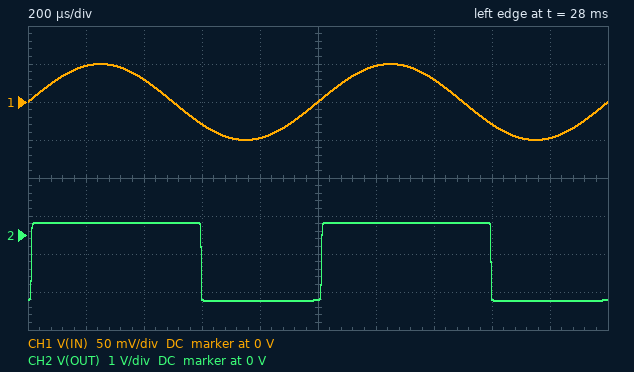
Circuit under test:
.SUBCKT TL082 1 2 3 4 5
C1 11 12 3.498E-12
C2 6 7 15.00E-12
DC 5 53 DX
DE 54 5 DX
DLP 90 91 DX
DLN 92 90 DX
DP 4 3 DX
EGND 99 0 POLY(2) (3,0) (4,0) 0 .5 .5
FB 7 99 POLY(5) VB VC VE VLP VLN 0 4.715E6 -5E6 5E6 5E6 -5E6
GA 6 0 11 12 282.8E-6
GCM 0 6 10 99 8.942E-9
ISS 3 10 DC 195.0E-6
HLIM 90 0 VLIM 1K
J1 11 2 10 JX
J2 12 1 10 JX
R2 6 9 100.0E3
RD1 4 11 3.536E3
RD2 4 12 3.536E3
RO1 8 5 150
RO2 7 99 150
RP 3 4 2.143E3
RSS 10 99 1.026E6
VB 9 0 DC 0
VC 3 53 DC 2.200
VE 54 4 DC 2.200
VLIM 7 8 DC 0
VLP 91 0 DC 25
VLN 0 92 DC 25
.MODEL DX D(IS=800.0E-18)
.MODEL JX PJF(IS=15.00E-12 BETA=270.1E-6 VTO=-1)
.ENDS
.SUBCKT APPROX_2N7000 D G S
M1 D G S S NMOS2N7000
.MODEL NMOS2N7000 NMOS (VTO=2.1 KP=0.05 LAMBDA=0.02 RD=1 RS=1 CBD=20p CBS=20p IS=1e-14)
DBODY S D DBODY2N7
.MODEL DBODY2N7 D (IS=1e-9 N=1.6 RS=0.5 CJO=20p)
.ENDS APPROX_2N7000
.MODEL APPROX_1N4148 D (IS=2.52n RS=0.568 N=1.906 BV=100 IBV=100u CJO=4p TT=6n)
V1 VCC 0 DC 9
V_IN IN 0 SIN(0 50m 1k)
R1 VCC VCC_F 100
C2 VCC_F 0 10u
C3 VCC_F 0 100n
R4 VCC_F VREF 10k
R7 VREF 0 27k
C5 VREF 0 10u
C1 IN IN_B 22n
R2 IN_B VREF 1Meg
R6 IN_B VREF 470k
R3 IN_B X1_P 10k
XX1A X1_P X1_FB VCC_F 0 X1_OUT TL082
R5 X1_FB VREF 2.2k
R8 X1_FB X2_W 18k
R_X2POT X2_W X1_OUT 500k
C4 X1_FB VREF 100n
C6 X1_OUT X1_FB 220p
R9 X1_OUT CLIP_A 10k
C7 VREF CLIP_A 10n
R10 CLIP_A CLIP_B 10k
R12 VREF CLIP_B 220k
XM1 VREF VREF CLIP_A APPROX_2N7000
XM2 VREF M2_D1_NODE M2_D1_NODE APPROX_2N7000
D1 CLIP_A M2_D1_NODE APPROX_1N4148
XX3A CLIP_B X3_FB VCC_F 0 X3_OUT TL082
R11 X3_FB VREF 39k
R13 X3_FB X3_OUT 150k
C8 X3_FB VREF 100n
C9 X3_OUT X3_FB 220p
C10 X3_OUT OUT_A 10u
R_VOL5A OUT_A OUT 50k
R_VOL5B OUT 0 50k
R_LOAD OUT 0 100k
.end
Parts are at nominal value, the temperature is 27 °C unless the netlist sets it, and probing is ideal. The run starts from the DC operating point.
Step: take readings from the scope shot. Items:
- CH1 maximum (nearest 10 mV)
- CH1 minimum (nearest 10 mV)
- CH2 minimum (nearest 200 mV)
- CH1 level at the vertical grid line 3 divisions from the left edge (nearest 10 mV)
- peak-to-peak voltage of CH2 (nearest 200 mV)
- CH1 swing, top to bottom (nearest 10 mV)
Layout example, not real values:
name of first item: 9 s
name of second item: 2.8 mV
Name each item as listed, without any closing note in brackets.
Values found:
CH1 maximum: 50 mV
CH1 minimum: -50 mV
CH2 minimum: -1.8 V
CH1 level at the vertical grid line 3 divisions from the left edge: -30 mV
peak-to-peak voltage of CH2: 2.0 V
CH1 swing, top to bottom: 100 mV
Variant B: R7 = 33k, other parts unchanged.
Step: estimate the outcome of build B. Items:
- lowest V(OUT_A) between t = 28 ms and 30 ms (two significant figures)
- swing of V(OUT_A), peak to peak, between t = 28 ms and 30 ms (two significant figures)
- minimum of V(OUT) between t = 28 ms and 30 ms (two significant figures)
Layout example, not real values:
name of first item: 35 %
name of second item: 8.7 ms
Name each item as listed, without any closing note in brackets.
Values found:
lowest V(OUT_A) between t = 28 ms and 30 ms: -4.6 V
swing of V(OUT_A), peak to peak, between t = 28 ms and 30 ms: 5.1 V
minimum of V(OUT) between t = 28 ms and 30 ms: -1.8 V
